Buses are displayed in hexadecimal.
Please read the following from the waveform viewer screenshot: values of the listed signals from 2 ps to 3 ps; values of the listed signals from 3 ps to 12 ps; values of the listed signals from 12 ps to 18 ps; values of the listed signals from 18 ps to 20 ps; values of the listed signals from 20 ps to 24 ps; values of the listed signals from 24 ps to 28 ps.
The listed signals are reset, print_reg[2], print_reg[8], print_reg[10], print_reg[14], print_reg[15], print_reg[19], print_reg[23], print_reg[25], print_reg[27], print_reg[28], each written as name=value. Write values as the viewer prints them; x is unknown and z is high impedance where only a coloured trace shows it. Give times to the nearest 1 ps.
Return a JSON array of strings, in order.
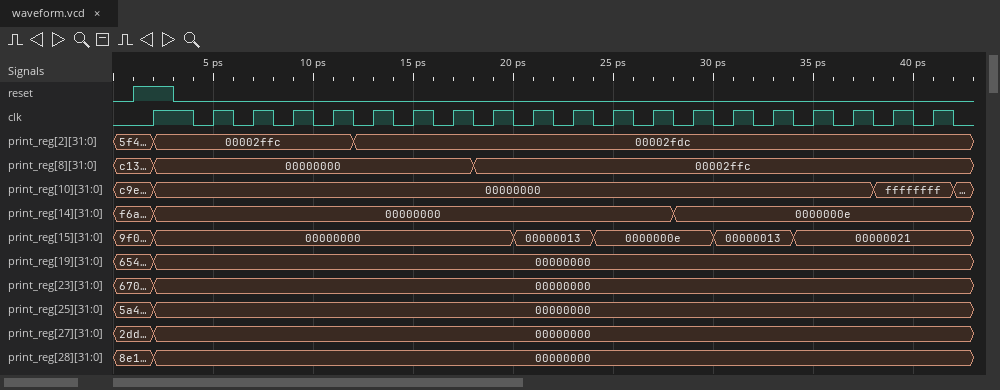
["reset=1, print_reg[2]=00002ffc, print_reg[8]=00000000, print_reg[10]=00000000, print_reg[14]=00000000, print_reg[15]=00000000, print_reg[19]=00000000, print_reg[23]=00000000, print_reg[25]=00000000, print_reg[27]=00000000, print_reg[28]=00000000", "reset=0, print_reg[2]=00002ffc, print_reg[8]=00000000, print_reg[10]=00000000, print_reg[14]=00000000, print_reg[15]=00000000, print_reg[19]=00000000, print_reg[23]=00000000, print_reg[25]=00000000, print_reg[27]=00000000, print_reg[28]=00000000", "reset=0, print_reg[2]=00002fdc, print_reg[8]=00000000, print_reg[10]=00000000, print_reg[14]=00000000, print_reg[15]=00000000, print_reg[19]=00000000, print_reg[23]=00000000, print_reg[25]=00000000, print_reg[27]=00000000, print_reg[28]=00000000", "reset=0, print_reg[2]=00002fdc, print_reg[8]=00002ffc, print_reg[10]=00000000, print_reg[14]=00000000, print_reg[15]=00000000, print_reg[19]=00000000, print_reg[23]=00000000, print_reg[25]=00000000, print_reg[27]=00000000, print_reg[28]=00000000", "reset=0, print_reg[2]=00002fdc, print_reg[8]=00002ffc, print_reg[10]=00000000, print_reg[14]=00000000, print_reg[15]=00000013, print_reg[19]=00000000, print_reg[23]=00000000, print_reg[25]=00000000, print_reg[27]=00000000, print_reg[28]=00000000", "reset=0, print_reg[2]=00002fdc, print_reg[8]=00002ffc, print_reg[10]=00000000, print_reg[14]=00000000, print_reg[15]=0000000e, print_reg[19]=00000000, print_reg[23]=00000000, print_reg[25]=00000000, print_reg[27]=00000000, print_reg[28]=00000000"]
